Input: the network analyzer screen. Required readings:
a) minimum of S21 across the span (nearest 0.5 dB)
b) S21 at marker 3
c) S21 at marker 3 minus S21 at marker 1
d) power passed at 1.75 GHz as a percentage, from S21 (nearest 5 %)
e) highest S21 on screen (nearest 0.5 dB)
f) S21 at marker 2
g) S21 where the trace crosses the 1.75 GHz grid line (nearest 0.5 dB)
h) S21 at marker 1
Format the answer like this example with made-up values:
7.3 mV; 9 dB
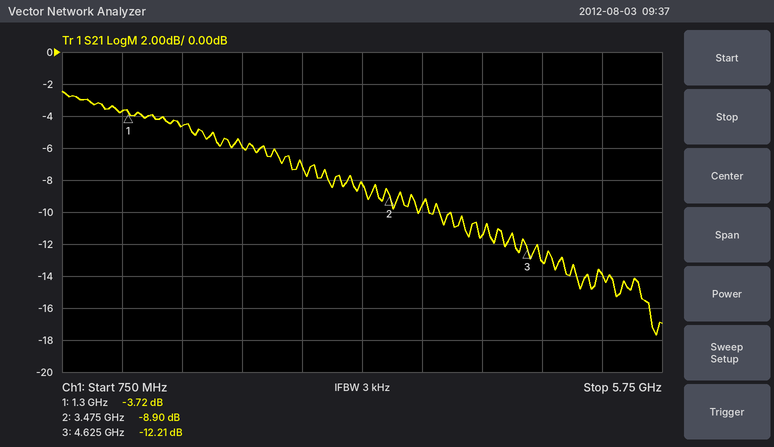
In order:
-17.5 dB; -12.21 dB; -8.49 dB; 35 %; -2.5 dB; -8.90 dB; -4.5 dB; -3.72 dB
